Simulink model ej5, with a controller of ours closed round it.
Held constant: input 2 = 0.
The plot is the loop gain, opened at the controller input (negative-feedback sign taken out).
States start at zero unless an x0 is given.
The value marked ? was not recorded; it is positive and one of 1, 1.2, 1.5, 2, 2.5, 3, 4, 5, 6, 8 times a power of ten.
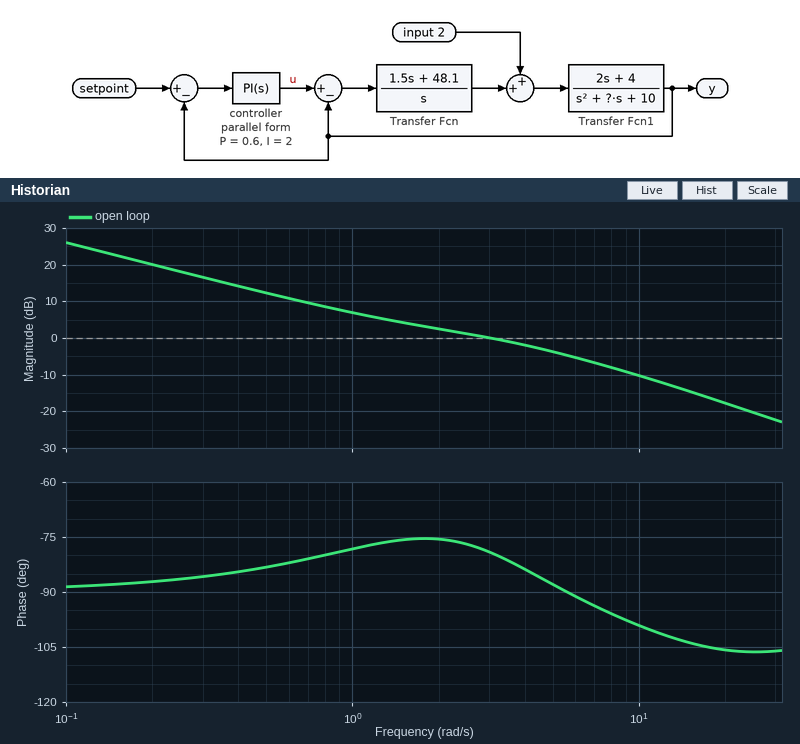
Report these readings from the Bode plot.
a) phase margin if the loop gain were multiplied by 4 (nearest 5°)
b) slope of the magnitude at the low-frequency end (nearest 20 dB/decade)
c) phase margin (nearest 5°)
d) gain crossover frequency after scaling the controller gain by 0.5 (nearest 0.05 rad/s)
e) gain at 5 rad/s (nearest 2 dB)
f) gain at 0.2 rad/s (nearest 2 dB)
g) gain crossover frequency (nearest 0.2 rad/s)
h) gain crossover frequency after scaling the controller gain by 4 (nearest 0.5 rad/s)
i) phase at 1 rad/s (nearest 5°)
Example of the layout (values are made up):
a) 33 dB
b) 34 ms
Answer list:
a) 80°
b) -20 dB/decade
c) 100°
d) 1.15 rad/s
e) -4 dB
f) 20 dB
g) 3.0 rad/s
h) 12.0 rad/s
i) -80°
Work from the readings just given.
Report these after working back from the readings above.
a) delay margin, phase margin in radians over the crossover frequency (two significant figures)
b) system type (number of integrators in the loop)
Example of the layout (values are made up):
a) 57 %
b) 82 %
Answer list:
a) 0.58 s
b) 1
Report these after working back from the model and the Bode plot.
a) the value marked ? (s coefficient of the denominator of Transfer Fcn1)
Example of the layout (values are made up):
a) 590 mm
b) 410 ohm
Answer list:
a) 20
